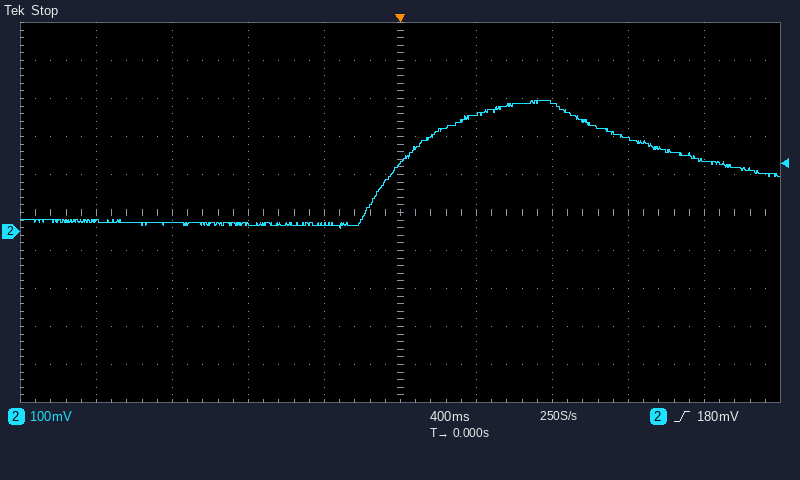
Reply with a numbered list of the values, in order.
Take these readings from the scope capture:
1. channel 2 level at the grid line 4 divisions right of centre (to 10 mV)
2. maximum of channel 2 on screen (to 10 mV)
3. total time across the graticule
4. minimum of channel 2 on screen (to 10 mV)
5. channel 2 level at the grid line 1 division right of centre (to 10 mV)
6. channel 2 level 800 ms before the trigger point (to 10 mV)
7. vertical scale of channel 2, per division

1. 190 mV
2. 340 mV
3. 4 s
4. 10 mV
5. 310 mV
6. 20 mV
7. 100 mV
